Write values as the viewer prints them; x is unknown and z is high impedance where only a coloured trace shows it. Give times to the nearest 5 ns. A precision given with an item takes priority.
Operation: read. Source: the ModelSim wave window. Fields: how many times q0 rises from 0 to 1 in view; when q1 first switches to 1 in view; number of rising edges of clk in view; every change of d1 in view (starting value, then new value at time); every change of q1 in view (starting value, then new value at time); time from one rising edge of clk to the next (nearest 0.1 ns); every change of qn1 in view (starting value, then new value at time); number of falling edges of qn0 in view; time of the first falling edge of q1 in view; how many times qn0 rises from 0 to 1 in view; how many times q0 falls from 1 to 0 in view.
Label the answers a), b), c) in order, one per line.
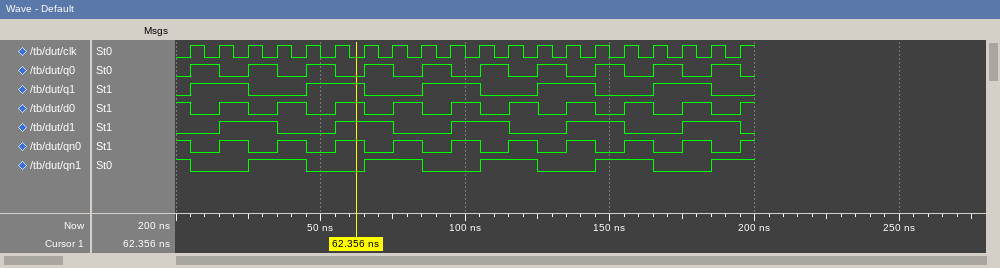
a) 10
b) 5 ns
c) 20
d) 0, 1 at 15 ns, 0 at 35 ns, 1 at 55 ns, 0 at 75 ns, 1 at 95 ns, 0 at 115 ns, 1 at 135 ns, 0 at 155 ns, 1 at 175 ns, 0 at 195 ns
e) 0, 1 at 5 ns, 0 at 25 ns, 1 at 45 ns, 0 at 65 ns, 1 at 85 ns, 0 at 105 ns, 1 at 125 ns, 0 at 145 ns, 1 at 165 ns, 0 at 185 ns
f) 10 ns
g) 1, 0 at 5 ns, 1 at 25 ns, 0 at 45 ns, 1 at 65 ns, 0 at 85 ns, 1 at 105 ns, 0 at 125 ns, 1 at 145 ns, 0 at 165 ns, 1 at 185 ns
h) 10
i) 25 ns
j) 10
k) 10
